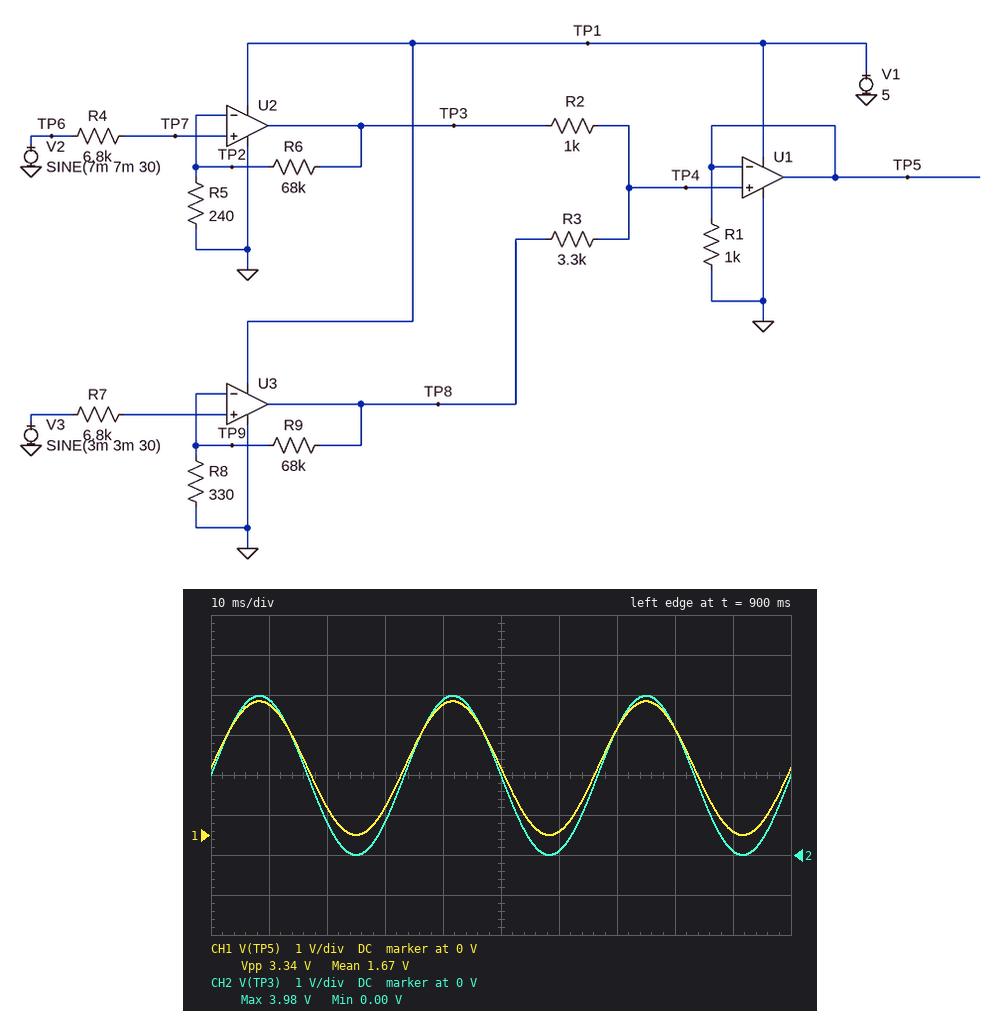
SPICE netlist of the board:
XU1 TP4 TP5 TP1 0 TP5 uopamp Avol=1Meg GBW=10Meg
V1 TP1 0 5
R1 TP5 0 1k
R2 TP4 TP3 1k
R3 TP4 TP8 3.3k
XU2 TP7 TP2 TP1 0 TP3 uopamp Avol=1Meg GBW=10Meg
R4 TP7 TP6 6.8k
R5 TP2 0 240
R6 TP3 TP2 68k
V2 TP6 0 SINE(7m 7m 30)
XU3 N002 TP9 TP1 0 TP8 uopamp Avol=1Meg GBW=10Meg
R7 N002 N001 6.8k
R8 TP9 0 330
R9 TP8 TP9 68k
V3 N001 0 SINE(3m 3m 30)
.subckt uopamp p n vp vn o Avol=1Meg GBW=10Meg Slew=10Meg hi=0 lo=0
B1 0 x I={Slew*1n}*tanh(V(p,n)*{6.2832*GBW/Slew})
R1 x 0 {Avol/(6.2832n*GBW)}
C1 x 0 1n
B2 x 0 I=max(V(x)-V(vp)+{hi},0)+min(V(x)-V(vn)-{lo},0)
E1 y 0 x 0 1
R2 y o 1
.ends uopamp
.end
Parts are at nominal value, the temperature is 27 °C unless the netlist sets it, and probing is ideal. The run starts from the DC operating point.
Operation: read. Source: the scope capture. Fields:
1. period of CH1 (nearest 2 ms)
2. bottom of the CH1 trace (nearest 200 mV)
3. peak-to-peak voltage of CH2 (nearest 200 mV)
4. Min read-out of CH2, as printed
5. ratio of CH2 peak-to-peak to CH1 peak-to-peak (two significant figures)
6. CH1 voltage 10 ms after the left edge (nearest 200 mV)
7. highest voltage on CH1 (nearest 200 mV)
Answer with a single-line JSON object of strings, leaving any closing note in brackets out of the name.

{"period of CH1": "34 ms", "bottom of the CH1 trace": "0 V", "peak-to-peak voltage of CH2": "4.0 V", "Min read-out of CH2, as printed": "0.00 V", "ratio of CH2 peak-to-peak to CH1 peak-to-peak": "1.2", "CH1 voltage 10 ms after the left edge": "3.2 V", "highest voltage on CH1": "3.4 V"}
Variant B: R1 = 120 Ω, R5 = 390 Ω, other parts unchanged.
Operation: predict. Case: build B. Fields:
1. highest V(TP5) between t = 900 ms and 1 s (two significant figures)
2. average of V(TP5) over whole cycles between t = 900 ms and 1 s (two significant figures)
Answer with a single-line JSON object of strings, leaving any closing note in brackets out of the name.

{"highest V(TP5) between t = 900 ms and 1 s": "2.2 V", "average of V(TP5) over whole cycles between t = 900 ms and 1 s": "1.1 V"}
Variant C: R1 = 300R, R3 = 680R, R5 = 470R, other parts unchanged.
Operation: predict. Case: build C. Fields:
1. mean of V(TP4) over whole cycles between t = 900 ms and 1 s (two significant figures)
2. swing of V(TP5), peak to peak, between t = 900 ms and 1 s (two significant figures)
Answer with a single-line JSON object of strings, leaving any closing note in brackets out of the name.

{"mean of V(TP4) over whole cycles between t = 900 ms and 1 s": "780 mV", "swing of V(TP5), peak to peak, between t = 900 ms and 1 s": "1.6 V"}
